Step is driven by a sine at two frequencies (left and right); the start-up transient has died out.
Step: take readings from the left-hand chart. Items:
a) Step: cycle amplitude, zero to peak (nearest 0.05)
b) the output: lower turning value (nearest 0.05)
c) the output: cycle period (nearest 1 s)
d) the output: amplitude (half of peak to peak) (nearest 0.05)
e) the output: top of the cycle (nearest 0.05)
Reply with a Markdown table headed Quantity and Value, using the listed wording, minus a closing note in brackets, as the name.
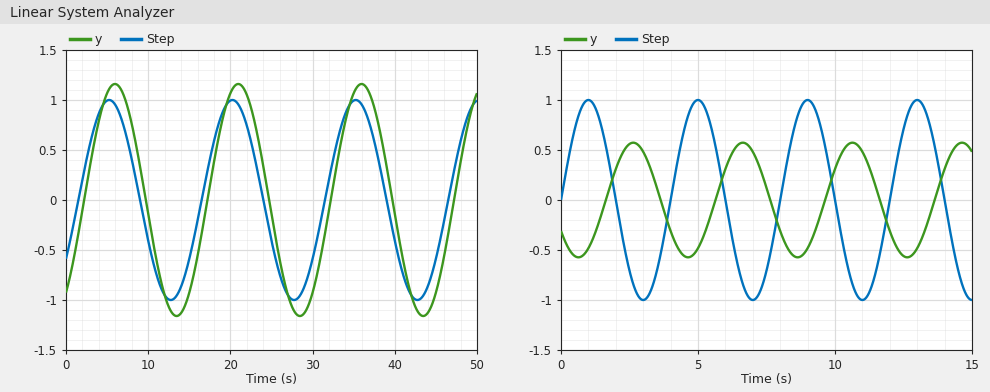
| Quantity | Value |
|---|---|
| Step: cycle amplitude, zero to peak | 1.00 |
| the output: lower turning value | -1.15 |
| the output: cycle period | 15 s |
| the output: amplitude (half of peak to peak) | 1.15 |
| the output: top of the cycle | 1.15 |
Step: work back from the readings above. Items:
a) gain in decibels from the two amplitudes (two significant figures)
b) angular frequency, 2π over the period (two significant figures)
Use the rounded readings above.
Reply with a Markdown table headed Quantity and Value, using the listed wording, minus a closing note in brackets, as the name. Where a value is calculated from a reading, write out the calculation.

| Quantity | Value |
|---|---|
| gain in decibels from the two amplitudes | 20 log10(1.15 / 1) = 1.2 dB |
| angular frequency, 2π over the period | 2π / 15 = 0.42 rad/s |
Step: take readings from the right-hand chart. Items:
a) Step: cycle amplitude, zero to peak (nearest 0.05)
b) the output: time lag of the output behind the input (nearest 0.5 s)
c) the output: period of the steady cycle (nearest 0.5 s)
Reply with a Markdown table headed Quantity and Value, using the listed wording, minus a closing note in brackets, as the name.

| Quantity | Value |
|---|---|
| Step: cycle amplitude, zero to peak | 1.00 |
| the output: time lag of the output behind the input | 1.5 s |
| the output: period of the steady cycle | 4.0 s |
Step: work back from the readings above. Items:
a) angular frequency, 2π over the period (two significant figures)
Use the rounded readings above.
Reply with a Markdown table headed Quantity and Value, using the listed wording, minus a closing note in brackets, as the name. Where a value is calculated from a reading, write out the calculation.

| Quantity | Value |
|---|---|
| angular frequency, 2π over the period | 2π / 4 = 1.6 rad/s |
